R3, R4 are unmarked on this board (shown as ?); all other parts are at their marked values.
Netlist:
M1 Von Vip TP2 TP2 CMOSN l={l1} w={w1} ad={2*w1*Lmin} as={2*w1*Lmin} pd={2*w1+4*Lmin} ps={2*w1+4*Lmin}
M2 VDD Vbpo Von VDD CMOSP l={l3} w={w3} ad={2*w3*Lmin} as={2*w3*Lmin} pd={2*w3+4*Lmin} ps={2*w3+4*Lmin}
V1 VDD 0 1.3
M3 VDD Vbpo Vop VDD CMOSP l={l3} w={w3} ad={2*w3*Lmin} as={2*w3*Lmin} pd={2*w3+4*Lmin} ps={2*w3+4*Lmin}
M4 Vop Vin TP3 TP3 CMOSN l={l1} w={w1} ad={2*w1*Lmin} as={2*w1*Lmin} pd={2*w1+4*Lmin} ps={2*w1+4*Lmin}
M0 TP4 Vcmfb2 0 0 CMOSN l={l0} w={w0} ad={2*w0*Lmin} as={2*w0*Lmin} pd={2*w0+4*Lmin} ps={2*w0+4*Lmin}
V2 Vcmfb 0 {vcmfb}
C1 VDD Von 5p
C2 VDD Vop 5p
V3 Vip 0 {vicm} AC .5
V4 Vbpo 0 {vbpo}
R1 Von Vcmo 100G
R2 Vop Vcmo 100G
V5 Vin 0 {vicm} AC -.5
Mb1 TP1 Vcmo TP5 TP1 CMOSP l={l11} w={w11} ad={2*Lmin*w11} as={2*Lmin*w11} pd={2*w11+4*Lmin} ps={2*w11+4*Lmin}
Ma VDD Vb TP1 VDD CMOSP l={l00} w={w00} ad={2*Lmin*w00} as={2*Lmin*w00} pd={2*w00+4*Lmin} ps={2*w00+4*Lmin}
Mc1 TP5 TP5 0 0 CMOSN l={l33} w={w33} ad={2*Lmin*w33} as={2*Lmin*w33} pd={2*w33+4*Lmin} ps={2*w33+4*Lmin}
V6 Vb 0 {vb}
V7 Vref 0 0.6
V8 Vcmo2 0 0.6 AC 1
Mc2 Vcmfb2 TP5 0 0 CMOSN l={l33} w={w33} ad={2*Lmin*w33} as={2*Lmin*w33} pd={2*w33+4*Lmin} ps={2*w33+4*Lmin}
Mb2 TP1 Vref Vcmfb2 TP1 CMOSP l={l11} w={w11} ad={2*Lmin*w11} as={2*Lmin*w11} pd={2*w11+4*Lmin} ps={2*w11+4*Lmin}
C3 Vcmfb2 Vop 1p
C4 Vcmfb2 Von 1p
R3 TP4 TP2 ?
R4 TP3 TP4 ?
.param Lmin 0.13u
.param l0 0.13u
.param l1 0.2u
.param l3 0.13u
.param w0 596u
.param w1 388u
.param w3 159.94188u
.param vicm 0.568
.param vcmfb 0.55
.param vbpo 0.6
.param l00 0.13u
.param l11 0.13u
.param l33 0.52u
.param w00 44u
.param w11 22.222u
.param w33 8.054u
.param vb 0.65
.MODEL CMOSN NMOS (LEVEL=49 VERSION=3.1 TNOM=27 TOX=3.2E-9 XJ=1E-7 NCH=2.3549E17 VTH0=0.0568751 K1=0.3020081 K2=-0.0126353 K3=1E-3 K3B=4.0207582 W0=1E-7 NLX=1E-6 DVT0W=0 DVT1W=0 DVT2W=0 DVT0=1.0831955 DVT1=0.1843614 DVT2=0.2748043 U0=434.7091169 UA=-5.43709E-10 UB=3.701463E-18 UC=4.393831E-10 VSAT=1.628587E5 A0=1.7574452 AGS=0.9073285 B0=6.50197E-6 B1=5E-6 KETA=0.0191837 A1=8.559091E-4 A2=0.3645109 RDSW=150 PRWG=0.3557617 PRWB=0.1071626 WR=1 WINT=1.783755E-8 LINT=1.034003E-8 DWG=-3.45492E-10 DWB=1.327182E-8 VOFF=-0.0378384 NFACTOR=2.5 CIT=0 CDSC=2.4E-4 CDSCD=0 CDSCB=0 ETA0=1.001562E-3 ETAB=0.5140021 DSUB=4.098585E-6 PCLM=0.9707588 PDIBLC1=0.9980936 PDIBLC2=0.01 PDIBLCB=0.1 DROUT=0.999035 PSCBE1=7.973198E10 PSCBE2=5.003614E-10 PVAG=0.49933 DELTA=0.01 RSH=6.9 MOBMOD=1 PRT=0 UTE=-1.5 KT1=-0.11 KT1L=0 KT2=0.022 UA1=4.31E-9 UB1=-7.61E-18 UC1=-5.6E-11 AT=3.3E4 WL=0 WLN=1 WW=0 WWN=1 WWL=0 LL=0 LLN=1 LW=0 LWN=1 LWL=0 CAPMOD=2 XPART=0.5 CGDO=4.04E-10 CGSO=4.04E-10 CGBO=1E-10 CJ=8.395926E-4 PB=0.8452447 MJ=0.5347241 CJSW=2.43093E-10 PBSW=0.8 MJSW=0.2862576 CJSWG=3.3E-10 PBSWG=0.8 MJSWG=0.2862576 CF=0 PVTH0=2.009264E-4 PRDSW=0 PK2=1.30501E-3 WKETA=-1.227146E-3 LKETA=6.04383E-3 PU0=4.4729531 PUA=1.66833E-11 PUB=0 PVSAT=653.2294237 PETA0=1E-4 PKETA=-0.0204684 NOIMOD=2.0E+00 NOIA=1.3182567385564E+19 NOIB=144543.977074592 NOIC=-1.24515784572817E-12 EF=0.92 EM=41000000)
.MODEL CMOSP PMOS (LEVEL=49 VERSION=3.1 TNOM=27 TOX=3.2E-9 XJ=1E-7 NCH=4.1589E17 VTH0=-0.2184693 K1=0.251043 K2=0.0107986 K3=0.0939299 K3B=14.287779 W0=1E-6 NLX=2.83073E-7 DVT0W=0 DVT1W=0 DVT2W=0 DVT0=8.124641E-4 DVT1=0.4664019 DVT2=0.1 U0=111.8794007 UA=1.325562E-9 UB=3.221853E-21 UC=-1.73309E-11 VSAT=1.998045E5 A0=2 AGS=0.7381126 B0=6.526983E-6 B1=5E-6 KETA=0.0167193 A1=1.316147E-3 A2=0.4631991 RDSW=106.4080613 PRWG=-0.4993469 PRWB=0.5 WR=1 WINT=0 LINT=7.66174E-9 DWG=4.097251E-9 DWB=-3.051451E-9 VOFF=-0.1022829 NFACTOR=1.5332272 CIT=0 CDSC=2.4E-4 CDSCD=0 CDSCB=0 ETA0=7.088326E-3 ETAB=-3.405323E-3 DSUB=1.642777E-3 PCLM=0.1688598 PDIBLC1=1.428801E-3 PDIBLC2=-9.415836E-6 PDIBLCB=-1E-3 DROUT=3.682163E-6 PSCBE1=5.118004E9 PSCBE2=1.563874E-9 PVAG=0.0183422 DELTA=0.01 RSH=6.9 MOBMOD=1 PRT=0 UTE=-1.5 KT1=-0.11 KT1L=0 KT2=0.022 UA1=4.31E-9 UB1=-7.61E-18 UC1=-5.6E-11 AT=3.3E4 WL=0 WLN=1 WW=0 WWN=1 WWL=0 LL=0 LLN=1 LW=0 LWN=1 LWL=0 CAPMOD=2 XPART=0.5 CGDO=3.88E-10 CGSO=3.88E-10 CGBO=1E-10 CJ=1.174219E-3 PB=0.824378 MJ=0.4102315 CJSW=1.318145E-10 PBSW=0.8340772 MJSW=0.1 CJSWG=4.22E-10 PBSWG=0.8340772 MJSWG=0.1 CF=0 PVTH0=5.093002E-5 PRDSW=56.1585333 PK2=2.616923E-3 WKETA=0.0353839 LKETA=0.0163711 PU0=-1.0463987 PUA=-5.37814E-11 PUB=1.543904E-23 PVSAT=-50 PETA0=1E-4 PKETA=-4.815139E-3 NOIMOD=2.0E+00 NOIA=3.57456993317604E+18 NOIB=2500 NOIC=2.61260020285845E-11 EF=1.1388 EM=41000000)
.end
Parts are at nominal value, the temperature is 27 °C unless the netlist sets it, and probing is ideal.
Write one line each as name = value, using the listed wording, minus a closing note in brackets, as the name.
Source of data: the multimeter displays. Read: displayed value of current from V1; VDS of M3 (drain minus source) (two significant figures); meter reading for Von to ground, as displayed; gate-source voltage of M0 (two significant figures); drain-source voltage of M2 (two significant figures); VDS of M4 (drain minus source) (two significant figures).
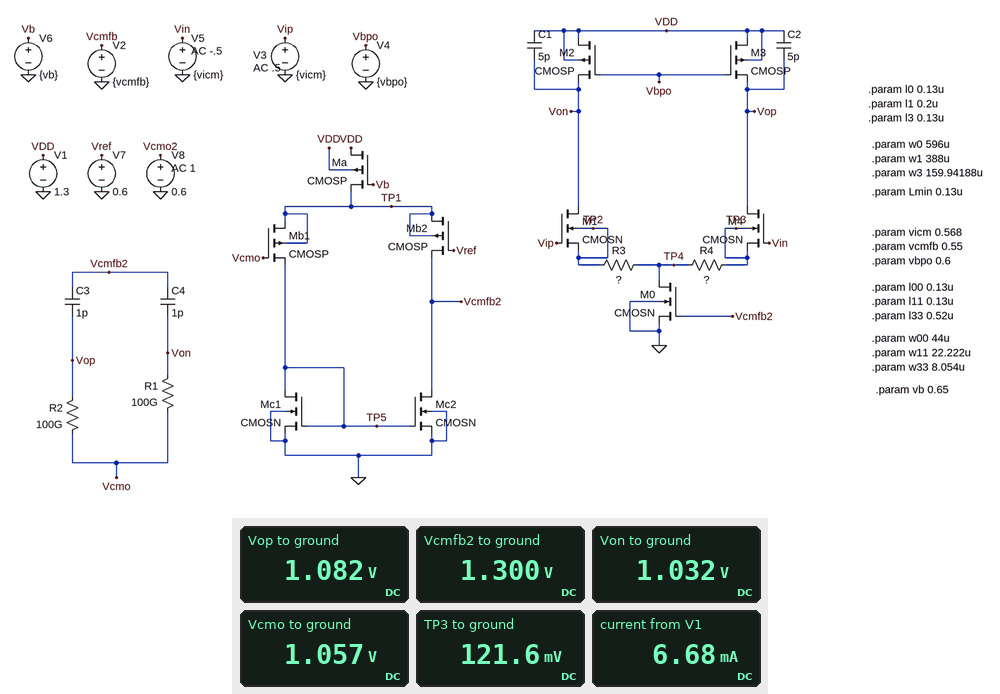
displayed value of current from V1 = 6.68 mA
VDS of M3 (drain minus source) = 220 mV
meter reading for Von to ground, as displayed = 1.032 V
gate-source voltage of M0 = 1.3 V
drain-source voltage of M2 = 270 mV
VDS of M4 (drain minus source) = 960 mV
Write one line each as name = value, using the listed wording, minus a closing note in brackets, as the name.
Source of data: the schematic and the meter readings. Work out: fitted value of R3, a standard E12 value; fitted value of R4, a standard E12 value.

fitted value of R3, a standard E12 value = 3.9 Ω
fitted value of R4, a standard E12 value = 6.8 Ω
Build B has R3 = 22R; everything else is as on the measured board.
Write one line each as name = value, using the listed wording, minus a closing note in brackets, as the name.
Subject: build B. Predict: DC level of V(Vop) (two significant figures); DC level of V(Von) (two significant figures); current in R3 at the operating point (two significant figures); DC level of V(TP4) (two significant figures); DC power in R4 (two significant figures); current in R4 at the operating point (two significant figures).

DC level of V(Vop) = 1.0 V
DC level of V(Von) = 1.2 V
current in R3 at the operating point = 2.4 mA
DC level of V(TP4) = 89 mV
DC power in R4 = 84 µW
current in R4 at the operating point = 3.5 mA
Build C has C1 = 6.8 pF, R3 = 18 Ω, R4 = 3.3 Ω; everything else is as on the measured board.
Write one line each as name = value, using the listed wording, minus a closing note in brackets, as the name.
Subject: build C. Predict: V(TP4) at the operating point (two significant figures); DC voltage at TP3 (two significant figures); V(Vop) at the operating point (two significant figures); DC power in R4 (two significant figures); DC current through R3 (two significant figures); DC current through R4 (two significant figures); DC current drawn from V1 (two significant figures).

V(TP4) at the operating point = 94 mV
DC voltage at TP3 = 110 mV
V(Vop) at the operating point = 940 mV
DC power in R4 = 46 µW
DC current through R3 = 2.5 mA
DC current through R4 = 3.7 mA
DC current drawn from V1 = 6.3 mA
